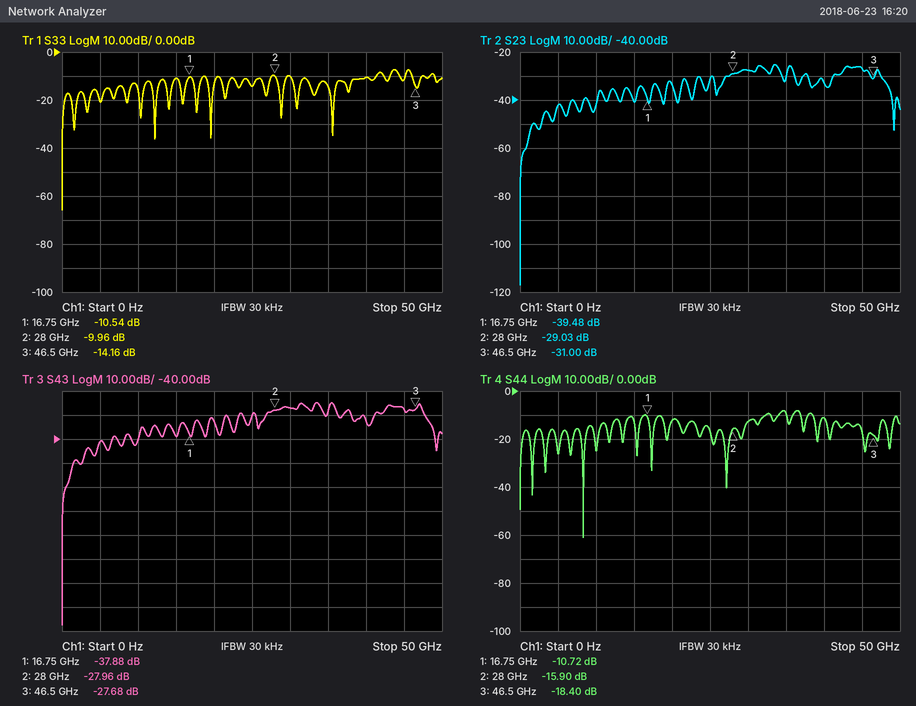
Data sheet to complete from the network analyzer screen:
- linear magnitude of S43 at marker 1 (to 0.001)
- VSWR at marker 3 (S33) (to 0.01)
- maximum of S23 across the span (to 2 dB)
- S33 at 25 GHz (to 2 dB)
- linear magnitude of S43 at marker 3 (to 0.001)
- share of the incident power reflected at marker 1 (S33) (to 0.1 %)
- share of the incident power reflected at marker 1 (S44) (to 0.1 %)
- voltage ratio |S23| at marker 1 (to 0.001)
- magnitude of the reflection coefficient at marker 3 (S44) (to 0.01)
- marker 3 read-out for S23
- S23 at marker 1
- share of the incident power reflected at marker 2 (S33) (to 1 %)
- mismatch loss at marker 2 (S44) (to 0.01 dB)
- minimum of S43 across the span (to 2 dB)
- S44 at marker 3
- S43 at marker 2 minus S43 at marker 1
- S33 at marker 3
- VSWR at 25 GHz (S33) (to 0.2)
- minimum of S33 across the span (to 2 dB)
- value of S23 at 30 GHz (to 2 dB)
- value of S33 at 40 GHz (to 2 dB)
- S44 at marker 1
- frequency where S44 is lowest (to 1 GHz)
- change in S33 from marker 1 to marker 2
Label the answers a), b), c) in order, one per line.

a) 0.013
b) 1.49
c) -26 dB
d) -14 dB
e) 0.041
f) 8.8 %
g) 8.5 %
h) 0.011
i) 0.12
j) -31.00 dB
k) -39.48 dB
l) 10 %
m) 0.11 dB
n) -118 dB
o) -18.40 dB
p) 9.92 dB
q) -14.16 dB
r) 1.4
s) -66 dB
t) -28 dB
u) -10 dB
v) -10.72 dB
w) 8 GHz
x) 0.58 dB
